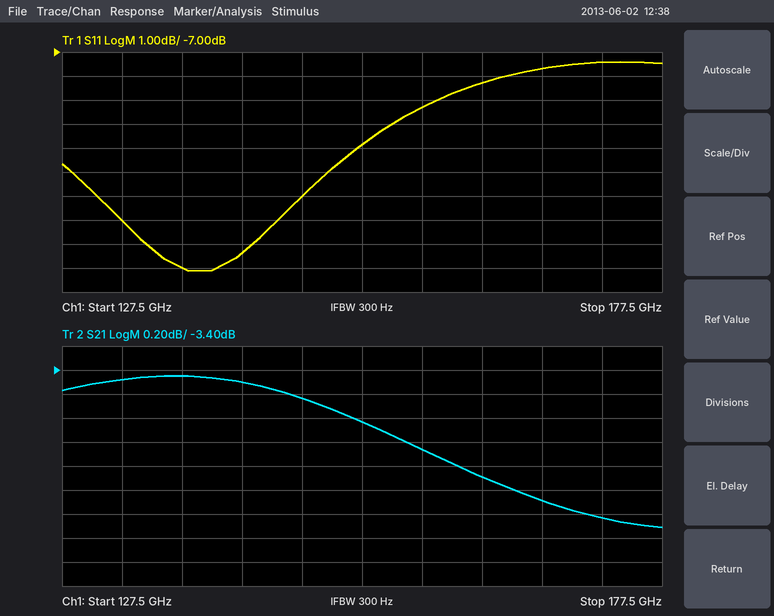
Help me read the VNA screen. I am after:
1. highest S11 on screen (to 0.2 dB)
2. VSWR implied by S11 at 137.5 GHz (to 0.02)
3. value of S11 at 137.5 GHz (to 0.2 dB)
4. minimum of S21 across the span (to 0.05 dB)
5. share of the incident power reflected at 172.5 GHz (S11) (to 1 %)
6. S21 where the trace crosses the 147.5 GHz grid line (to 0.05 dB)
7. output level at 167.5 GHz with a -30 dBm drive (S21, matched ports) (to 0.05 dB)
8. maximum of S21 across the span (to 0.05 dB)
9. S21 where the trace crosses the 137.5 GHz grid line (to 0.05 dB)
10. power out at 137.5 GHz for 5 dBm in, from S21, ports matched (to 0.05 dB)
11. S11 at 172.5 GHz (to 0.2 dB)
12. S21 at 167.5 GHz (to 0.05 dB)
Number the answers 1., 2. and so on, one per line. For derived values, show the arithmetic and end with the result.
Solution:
1. -7.4 dB
2. |Γ| = 10^(-16/20) = 0.1585; VSWR = (1 + 0.1585)/(1 − 0.1585) ≈ 1.38
3. -16.0 dB
4. -4.70 dB
5. 10^(-7.4/10) ≈ 18 %
6. -3.65 dB
7. -30 dBm + (-4.50 dB) = -34.50 dBm
8. -3.45 dB
9. -3.45 dB
10. 5 dBm + (-3.45 dB) = 1.55 dBm
11. -7.4 dB
12. -4.50 dB
